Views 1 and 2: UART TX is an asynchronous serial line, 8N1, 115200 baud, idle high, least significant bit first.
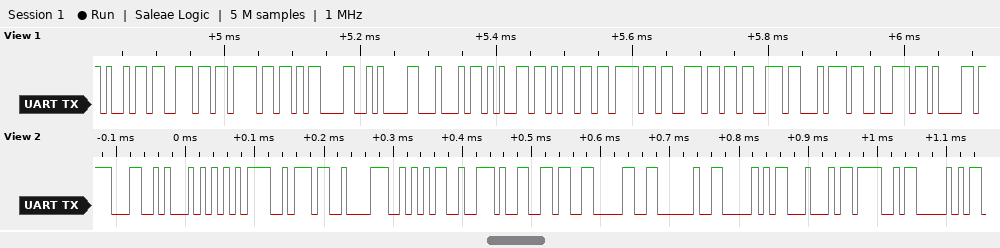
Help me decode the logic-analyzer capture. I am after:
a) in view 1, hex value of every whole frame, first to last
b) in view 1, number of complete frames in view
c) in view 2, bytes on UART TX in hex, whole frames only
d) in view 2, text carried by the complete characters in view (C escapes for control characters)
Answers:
0x69 0x6E 0x6F 0x0D 0x0A 0x44 0x65 0x6D 0x6F 0x6E 0x73 0x74 0x72 0x61
14
4C 54 3D 37 38 35 2E 36 30 20 50 44 4F 50
"LT=785.60 PDOP"
